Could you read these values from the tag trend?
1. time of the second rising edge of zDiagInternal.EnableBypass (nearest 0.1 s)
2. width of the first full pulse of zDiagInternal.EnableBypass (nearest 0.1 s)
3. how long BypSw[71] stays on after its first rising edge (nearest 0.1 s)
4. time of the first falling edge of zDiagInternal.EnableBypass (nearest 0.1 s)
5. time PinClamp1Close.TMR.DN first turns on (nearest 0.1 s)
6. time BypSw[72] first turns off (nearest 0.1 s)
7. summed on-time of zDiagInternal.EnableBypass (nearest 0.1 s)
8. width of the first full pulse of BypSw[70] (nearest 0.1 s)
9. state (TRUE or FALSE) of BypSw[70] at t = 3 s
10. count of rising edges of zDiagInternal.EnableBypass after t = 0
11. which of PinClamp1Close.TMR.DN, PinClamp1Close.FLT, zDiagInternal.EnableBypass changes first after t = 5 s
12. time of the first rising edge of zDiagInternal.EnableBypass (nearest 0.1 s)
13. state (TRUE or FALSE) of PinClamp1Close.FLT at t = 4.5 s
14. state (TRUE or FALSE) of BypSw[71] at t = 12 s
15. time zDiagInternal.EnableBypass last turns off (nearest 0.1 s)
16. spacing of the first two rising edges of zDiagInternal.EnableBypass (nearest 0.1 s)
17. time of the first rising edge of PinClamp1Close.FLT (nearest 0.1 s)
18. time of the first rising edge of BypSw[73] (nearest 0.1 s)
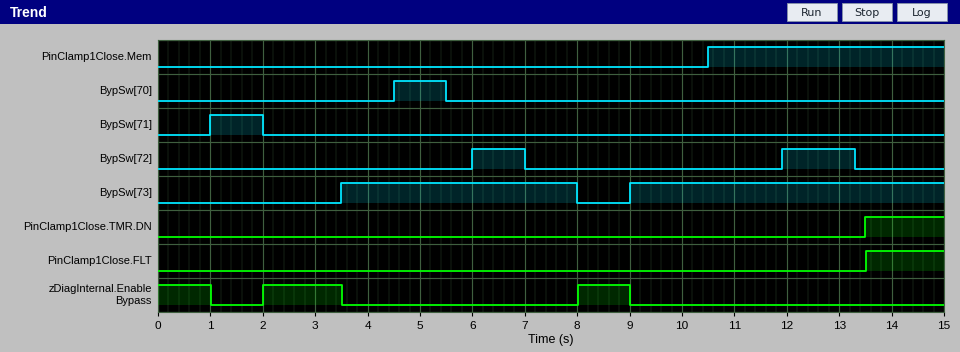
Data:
8.0 s
1.5 s
1.0 s
1.0 s
13.5 s
7.0 s
3.5 s
1.0 s
FALSE
2
zDiagInternal.EnableBypass
2.0 s
FALSE
FALSE
9.0 s
6.0 s
13.5 s
3.5 s
